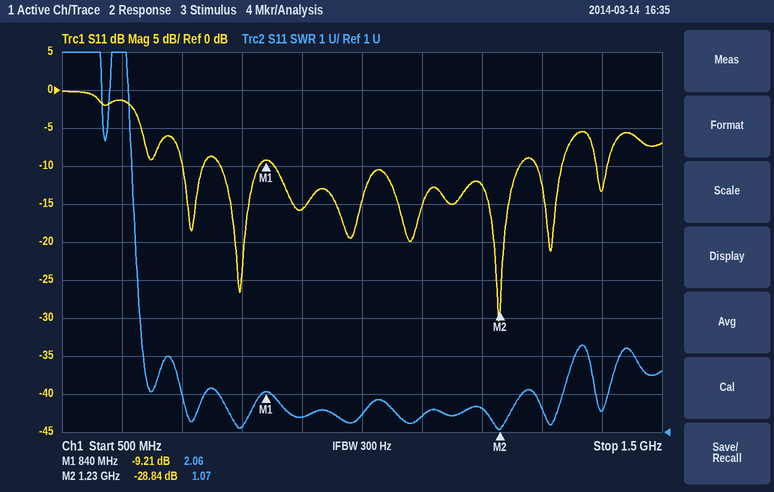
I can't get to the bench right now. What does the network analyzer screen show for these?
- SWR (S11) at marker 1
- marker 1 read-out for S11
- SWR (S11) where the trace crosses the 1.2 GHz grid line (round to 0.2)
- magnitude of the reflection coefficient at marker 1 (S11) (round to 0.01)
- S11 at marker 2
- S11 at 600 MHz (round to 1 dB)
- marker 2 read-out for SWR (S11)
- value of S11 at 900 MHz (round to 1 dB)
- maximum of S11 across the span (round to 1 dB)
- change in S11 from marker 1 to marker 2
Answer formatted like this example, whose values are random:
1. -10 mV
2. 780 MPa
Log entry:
1. 2.06
2. -9.21 dB
3. 1.6
4. 0.35
5. -28.84 dB
6. -1 dB
7. 1.07
8. -16 dB
9. 0 dB
10. -19.63 dB
